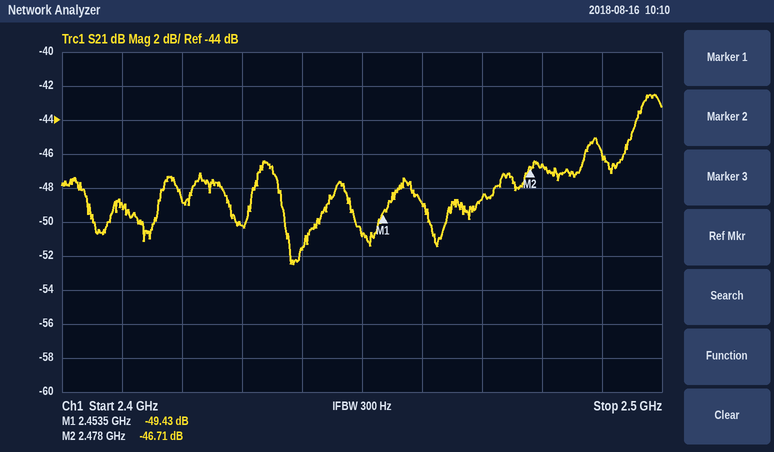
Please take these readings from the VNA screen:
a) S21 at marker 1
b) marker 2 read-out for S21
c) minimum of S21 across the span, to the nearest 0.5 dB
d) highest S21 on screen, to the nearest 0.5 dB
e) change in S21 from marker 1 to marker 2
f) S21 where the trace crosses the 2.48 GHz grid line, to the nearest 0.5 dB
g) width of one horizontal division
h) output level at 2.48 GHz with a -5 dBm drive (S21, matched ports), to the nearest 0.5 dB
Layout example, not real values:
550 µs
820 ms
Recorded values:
-49.43 dB
-46.71 dB
-52.5 dB
-42.5 dB
2.72 dB
-46.5 dB
10 MHz
-51.5 dBm
